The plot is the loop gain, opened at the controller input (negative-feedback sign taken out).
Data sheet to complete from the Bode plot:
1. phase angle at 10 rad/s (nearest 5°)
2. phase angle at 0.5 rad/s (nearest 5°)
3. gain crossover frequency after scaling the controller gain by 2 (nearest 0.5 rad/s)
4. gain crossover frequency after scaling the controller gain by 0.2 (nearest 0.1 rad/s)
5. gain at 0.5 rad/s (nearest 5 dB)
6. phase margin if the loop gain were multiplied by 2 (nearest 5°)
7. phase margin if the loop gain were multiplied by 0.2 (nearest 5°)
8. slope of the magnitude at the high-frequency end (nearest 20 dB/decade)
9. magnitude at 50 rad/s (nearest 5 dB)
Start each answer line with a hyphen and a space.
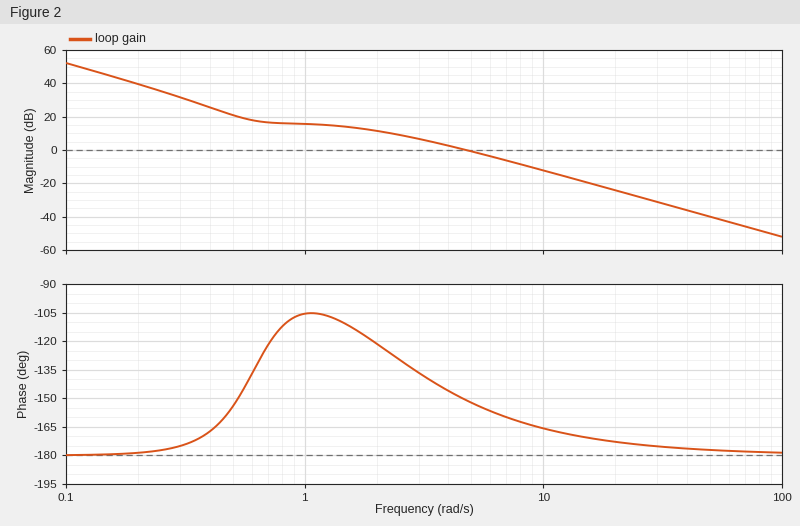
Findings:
- -165°
- -155°
- 7.0 rad/s
- 1.5 rad/s
- 20 dB
- 20°
- 70°
- -40 dB/decade
- -40 dB
